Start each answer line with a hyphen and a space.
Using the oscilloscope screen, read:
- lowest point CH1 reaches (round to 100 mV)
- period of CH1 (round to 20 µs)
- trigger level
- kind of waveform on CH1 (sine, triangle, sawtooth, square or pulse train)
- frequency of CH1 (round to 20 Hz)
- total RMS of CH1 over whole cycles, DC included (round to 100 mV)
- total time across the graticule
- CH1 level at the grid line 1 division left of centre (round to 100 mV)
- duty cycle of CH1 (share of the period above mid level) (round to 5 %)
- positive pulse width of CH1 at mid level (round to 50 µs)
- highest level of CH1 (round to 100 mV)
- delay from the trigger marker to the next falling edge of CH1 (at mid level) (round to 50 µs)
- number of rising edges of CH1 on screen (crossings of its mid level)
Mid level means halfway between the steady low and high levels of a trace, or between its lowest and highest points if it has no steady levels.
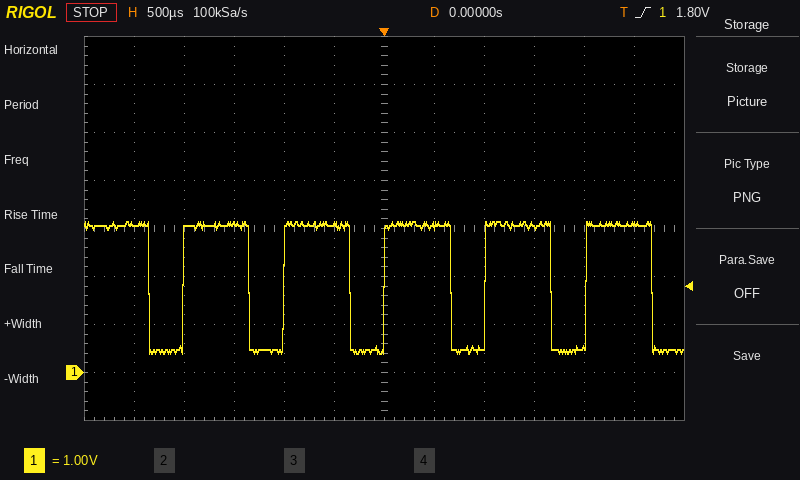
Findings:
- 400 mV
- 1.00 ms
- 1.80 V
- pulse train
- 1.00 kHz
- 2.5 V
- 6 ms
- 3.1 V
- 65 %
- 650 µs
- 3.1 V
- 650 µs
- 5
